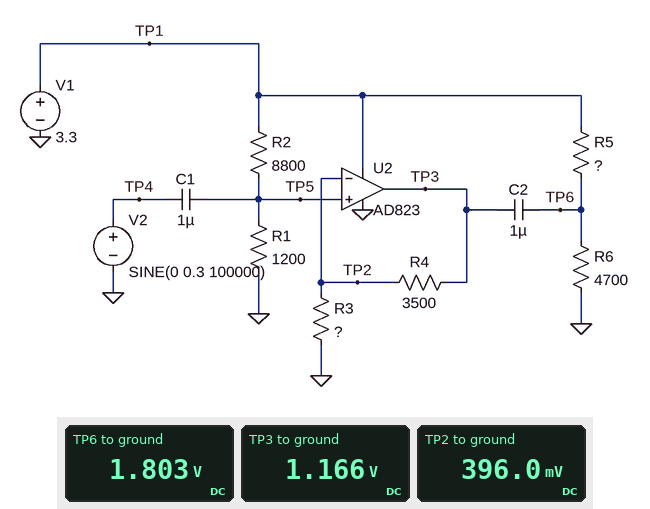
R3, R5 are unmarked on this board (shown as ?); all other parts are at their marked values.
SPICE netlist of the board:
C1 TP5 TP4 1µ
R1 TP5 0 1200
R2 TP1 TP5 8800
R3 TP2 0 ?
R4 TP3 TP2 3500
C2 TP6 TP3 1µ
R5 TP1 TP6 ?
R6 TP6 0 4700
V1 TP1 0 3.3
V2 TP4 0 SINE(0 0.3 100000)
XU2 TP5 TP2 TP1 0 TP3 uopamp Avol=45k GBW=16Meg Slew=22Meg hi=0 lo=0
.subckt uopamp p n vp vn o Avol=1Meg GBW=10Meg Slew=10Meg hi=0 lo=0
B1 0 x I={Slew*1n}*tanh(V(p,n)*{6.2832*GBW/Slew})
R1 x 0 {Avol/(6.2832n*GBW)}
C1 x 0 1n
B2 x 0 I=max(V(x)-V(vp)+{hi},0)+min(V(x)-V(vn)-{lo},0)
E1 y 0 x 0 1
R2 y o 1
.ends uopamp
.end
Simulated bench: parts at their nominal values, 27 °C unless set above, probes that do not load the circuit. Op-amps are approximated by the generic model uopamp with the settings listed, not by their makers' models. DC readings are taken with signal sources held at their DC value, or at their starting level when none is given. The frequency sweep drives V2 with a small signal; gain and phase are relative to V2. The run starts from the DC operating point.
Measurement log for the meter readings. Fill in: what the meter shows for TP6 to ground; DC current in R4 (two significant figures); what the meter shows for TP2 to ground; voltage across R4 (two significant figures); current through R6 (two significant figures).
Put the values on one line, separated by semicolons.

1.803 V; 220 µA; 396.0 mV; 770 mV; 380 µA
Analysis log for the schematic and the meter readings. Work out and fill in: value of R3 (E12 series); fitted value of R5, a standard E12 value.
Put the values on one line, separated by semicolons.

1.8 kΩ; 3.9 kΩ
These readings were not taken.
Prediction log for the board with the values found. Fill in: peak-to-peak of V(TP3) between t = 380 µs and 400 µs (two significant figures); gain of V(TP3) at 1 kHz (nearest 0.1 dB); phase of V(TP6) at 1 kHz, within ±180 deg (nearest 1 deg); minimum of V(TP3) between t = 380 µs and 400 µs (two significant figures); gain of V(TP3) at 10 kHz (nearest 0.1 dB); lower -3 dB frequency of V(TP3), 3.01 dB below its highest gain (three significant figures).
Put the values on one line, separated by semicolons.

1.8 V; 9.3 dB; 13 deg; 280 mV; 9.4 dB; 151 Hz
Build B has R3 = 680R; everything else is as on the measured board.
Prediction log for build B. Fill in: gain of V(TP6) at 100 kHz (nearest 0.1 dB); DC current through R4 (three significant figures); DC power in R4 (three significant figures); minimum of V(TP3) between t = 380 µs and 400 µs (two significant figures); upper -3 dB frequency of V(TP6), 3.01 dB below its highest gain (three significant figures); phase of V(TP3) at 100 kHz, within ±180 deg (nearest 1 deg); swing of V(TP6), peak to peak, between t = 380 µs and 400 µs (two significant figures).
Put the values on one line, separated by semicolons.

15.8 dB; 582 µA; 1.19 mW; 590 mV; 2.60 MHz; -2 deg; 2.7 V
